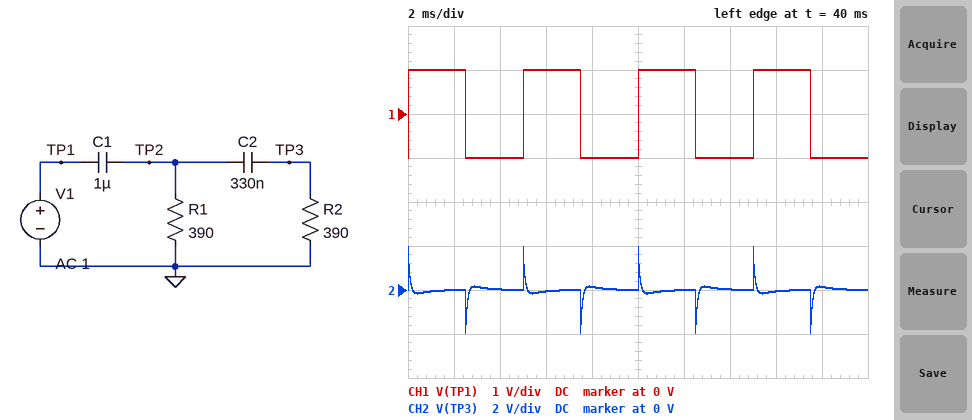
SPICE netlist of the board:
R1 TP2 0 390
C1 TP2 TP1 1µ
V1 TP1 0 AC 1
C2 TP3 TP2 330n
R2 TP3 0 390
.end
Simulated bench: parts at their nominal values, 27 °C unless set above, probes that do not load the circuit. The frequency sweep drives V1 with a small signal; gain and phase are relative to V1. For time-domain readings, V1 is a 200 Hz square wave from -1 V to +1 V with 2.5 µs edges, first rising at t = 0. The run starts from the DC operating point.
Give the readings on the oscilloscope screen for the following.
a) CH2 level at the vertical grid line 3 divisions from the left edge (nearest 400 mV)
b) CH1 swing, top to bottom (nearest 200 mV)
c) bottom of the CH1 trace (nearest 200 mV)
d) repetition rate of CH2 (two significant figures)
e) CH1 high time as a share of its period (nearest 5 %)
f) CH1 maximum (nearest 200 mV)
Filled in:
0 V
2.0 V
-1.0 V
200 Hz
50 %
1.0 V
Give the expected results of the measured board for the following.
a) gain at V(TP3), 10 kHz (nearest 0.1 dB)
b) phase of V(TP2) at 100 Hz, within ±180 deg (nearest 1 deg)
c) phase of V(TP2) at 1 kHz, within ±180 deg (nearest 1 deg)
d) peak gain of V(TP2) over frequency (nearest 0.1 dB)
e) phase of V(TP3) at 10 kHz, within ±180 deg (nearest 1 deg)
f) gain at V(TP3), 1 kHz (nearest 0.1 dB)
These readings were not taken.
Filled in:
-0.1 dB
72 deg
25 deg
0 dB
12 deg
-6.5 dB
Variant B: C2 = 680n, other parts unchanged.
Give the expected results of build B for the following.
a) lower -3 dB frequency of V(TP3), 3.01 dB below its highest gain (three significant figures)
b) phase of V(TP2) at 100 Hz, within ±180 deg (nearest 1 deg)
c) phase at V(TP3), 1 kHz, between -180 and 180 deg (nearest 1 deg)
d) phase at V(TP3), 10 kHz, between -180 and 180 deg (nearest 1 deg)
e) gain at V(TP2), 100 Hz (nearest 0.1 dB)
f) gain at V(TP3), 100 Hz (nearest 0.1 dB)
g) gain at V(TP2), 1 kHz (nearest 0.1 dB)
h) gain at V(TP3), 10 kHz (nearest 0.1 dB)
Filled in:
1.25 kHz
68 deg
62 deg
8 deg
-13.1 dB
-28.8 dB
-2.8 dB
-0.1 dB
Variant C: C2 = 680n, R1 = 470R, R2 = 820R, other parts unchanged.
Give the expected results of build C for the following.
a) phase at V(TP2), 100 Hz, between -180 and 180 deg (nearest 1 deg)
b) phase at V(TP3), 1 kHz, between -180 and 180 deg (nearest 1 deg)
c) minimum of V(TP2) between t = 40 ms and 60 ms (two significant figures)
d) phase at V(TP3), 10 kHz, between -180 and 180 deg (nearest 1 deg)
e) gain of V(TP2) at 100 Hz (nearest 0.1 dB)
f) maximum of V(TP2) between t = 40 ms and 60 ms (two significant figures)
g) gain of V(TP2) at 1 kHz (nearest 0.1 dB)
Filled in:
66 deg
42 deg
-1.9 V
5 deg
-11.9 dB
1.9 V
-1.4 dB
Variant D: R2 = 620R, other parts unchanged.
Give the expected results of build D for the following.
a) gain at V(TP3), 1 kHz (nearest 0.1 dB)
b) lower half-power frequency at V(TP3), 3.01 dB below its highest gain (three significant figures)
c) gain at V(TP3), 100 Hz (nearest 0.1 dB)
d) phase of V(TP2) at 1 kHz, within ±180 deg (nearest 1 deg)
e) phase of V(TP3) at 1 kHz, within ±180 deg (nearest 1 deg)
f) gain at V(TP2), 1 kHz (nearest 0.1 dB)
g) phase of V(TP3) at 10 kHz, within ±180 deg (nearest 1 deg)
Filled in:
-4.1 dB
1.23 kHz
-30.6 dB
27 deg
65 deg
-2.0 dB
8 deg
